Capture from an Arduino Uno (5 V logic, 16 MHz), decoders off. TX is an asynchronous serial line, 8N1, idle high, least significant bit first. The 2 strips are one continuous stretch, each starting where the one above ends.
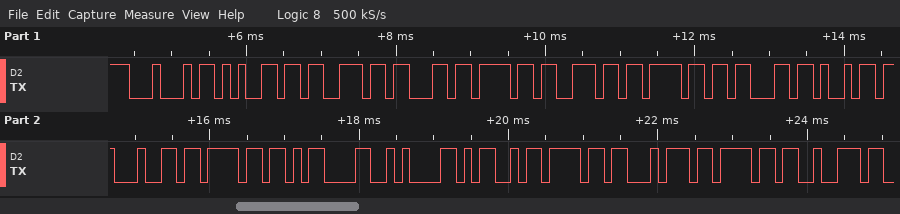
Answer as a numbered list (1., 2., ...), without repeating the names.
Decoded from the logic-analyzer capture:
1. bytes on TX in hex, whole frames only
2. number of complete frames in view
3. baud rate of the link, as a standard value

1. 0x44 0x65 0x73 0x63 0x6F 0x6E 0x6F 0x63 0x69 0x64 0x6F 0x0D 0x0A 0x4D 0x6F 0x74 0x6F 0x72
2. 18
3. 9600 baud
